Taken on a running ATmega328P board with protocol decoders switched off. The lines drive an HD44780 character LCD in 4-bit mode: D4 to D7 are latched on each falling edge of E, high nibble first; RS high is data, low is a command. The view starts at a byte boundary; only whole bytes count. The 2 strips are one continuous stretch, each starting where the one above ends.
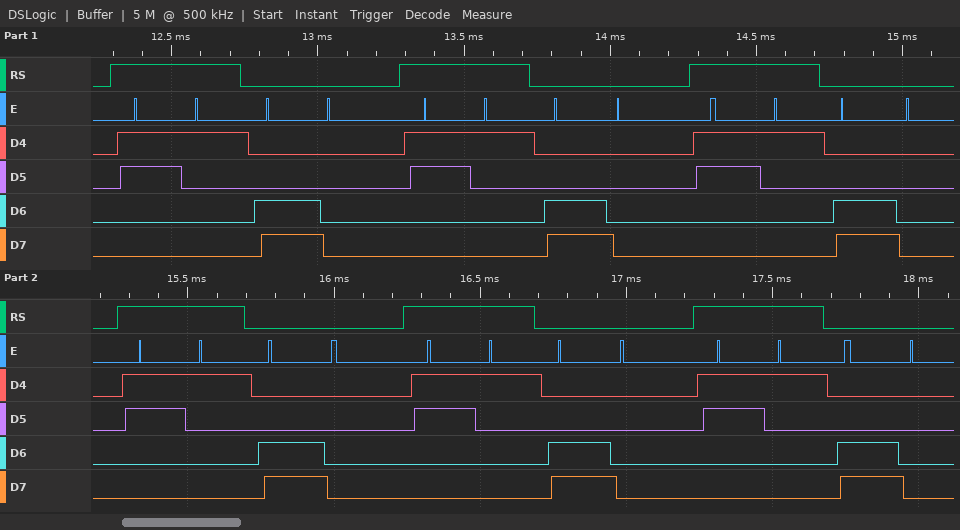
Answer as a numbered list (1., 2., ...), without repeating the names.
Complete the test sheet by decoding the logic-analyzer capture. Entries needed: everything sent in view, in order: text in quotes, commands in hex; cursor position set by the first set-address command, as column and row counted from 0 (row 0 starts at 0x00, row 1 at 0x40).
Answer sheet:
1. "1" 0xC0 "1" 0xC0 "1" 0xC0 "1" 0xC0 "1" 0xC0 "1" 0xC0
2. column 0, row 1
